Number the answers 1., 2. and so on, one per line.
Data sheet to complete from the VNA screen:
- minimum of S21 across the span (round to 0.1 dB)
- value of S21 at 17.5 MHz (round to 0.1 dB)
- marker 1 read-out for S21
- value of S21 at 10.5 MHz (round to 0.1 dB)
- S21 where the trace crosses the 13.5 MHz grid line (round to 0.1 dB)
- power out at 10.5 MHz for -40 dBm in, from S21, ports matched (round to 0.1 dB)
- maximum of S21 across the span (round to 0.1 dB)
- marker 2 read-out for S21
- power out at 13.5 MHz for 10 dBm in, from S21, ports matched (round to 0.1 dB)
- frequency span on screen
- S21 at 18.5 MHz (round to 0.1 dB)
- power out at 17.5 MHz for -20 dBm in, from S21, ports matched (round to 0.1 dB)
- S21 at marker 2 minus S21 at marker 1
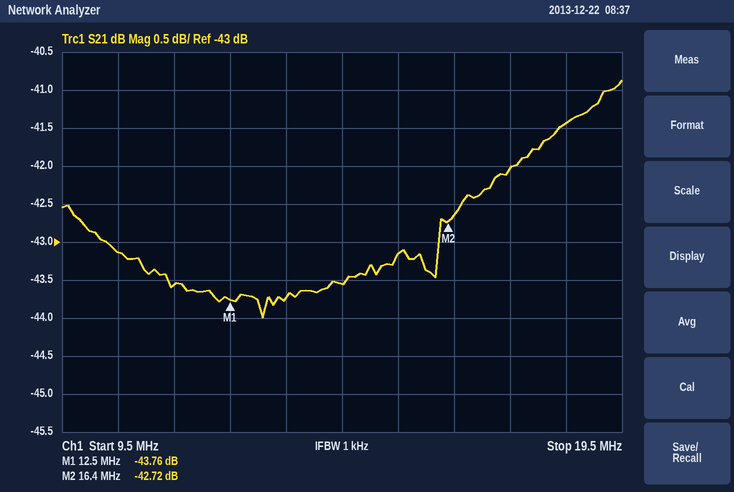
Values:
1. -44.0 dB
2. -42.0 dB
3. -43.76 dB
4. -43.1 dB
5. -43.7 dB
6. -83.1 dBm
7. -40.9 dB
8. -42.72 dB
9. -33.7 dBm
10. 10 MHz
11. -41.4 dB
12. -62.0 dBm
13. 1.04 dB
